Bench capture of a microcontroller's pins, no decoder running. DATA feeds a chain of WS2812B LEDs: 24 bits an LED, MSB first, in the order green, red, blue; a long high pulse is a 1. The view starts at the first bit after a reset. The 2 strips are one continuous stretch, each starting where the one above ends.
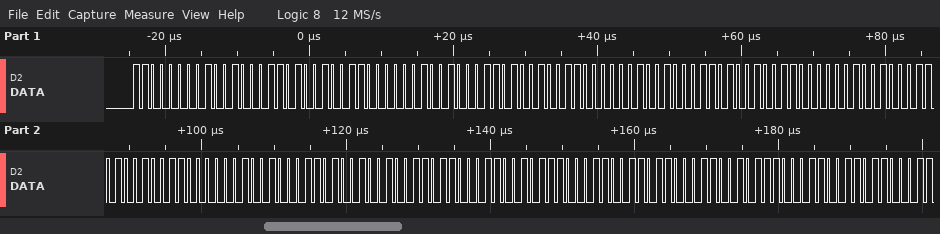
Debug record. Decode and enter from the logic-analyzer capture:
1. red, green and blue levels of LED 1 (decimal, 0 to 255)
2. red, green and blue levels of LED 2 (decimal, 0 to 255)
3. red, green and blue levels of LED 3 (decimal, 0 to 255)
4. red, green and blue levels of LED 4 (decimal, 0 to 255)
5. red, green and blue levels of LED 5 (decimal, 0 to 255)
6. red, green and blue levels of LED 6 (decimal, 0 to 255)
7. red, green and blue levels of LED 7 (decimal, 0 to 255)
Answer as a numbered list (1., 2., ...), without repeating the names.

1. 145, 192, 164
2. 145, 192, 164
3. 145, 192, 164
4. 145, 192, 164
5. 145, 192, 164
6. 25, 155, 113
7. 25, 155, 113
